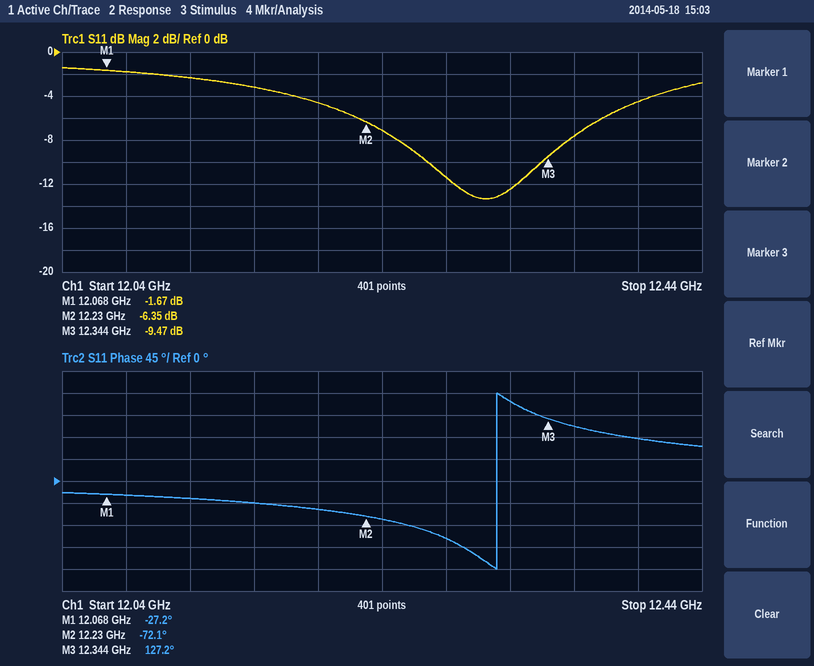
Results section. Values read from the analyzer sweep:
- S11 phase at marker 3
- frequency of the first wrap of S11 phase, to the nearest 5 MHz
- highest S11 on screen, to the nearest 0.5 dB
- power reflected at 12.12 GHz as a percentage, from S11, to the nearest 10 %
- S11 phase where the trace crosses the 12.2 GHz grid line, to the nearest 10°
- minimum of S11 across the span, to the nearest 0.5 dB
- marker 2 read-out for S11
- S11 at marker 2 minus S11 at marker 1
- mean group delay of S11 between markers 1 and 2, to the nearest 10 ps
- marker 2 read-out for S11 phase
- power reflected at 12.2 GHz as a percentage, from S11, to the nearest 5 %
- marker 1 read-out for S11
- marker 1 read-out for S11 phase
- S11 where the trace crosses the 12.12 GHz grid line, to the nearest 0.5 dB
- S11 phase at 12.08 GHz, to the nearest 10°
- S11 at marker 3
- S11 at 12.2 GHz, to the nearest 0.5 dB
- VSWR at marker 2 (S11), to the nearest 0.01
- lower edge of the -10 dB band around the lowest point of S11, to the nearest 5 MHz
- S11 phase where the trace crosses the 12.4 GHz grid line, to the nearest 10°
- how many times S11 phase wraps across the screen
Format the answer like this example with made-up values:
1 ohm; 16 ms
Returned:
127.2°; 12.310 GHz; -1.5 dB; 60 %; -60°; -13.5 dB; -6.35 dB; -4.68 dB; 770 ps; -72.1°; 35 %; -1.67 dB; -27.2°; -2.5 dB; -30°; -9.47 dB; -4.5 dB; 2.86; 12.270 GHz; 90°; 1
